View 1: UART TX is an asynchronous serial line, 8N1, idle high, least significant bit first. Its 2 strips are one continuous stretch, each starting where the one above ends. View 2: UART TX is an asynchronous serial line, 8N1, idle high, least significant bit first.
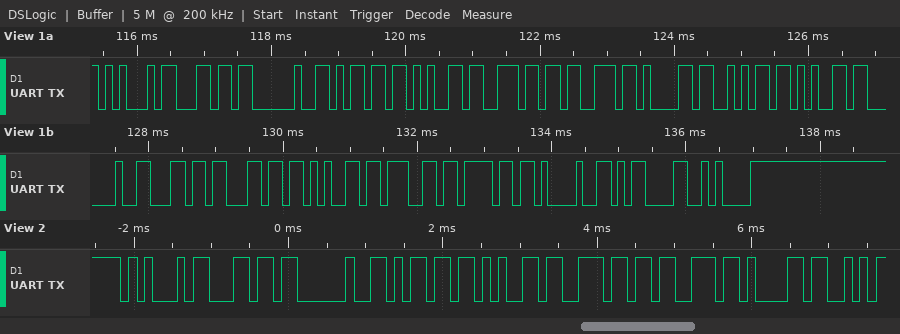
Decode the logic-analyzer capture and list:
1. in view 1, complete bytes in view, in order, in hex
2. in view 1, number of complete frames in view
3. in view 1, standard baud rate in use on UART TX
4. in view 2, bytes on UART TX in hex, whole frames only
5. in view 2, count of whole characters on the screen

45 6C 20 6D 65 6E 73 61 6A 65 20 6C 6C 65 67 6F 21 0D 0A
19
9600 baud
45 6C 20 6D 65 6E 73 61
8
